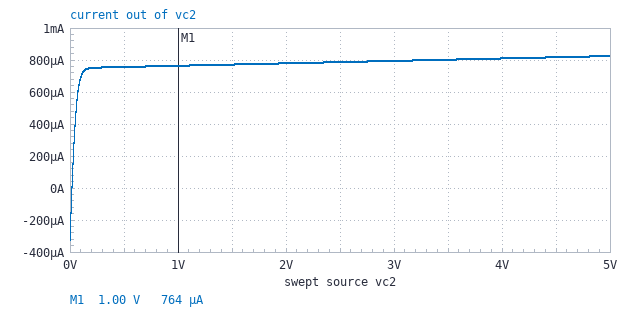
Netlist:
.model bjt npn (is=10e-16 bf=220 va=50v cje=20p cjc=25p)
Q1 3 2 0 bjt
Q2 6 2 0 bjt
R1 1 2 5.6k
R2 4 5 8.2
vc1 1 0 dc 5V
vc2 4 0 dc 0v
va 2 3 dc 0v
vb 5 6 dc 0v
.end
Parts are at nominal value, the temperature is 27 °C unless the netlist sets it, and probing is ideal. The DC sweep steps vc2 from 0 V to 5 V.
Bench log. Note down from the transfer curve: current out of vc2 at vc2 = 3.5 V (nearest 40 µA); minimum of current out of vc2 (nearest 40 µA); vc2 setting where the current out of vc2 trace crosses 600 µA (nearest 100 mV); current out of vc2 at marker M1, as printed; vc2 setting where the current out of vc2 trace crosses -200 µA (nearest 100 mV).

800 µA
-320 µA
100 mV
764 µA
0 V
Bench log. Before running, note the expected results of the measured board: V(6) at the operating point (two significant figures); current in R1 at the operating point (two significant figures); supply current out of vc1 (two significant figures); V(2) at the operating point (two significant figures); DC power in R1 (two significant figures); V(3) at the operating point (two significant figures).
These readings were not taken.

2.7 mV
770 µA
770 µA
690 mV
3.3 mW
690 mV
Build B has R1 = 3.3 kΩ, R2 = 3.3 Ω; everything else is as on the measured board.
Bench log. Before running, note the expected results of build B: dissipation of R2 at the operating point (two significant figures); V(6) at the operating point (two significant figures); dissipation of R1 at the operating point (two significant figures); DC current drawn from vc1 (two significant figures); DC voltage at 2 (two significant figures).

1.1 µW
1.9 mV
5.6 mW
1.3 mA
700 mV
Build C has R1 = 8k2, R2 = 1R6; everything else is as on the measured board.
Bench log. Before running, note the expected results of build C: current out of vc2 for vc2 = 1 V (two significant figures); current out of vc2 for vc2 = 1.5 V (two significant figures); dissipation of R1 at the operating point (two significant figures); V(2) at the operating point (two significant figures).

520 µA
530 µA
2.3 mW
680 mV
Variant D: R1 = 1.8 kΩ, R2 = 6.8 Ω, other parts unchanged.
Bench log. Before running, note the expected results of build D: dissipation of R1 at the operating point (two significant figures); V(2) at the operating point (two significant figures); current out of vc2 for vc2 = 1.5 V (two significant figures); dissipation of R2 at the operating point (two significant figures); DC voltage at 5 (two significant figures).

10 mW
720 mV
2.4 mA
4.5 µW
5.5 mV
